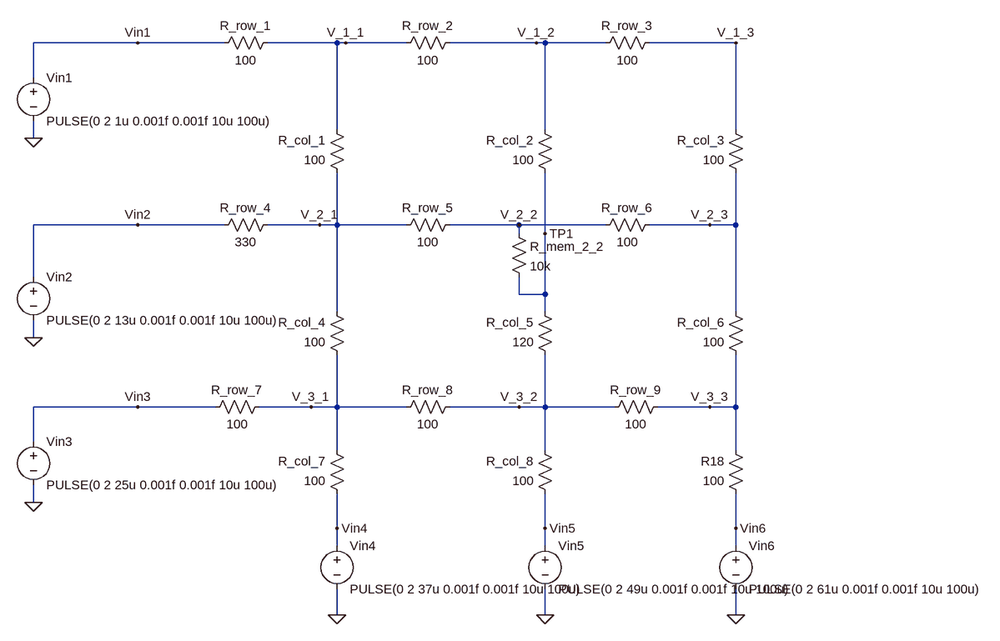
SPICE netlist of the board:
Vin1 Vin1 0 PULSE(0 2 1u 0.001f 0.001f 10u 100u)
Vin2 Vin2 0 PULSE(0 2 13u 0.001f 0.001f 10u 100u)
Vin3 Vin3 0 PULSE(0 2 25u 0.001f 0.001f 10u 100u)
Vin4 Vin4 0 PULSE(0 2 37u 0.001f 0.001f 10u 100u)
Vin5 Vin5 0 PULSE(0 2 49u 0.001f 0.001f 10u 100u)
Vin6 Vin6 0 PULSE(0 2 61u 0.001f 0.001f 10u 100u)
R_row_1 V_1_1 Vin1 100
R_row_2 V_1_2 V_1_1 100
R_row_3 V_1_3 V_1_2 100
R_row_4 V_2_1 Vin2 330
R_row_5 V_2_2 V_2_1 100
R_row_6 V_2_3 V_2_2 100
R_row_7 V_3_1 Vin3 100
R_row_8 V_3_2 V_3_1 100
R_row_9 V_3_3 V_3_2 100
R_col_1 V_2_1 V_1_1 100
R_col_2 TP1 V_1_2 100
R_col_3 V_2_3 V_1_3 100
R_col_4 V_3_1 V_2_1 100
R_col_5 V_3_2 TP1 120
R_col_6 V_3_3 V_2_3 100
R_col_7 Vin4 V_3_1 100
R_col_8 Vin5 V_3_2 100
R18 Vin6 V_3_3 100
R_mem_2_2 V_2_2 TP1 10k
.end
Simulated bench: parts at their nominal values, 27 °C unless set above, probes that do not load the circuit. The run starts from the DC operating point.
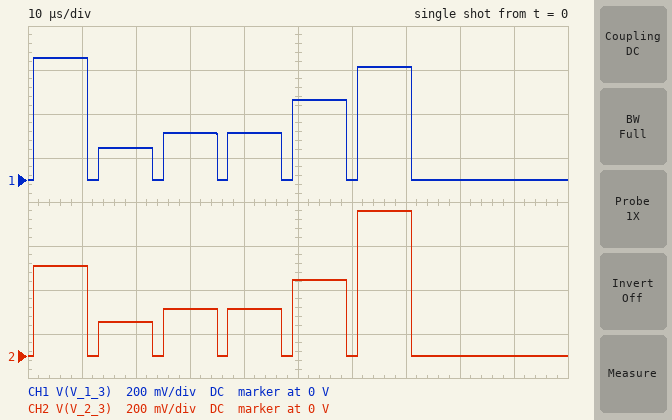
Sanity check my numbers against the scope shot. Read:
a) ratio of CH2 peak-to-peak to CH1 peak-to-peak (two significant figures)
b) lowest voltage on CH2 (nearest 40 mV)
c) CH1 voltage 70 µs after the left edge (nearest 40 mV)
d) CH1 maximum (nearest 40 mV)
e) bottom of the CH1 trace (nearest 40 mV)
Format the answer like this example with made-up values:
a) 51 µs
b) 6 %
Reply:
a) 1.2
b) 0 V
c) 520 mV
d) 560 mV
e) 0 V
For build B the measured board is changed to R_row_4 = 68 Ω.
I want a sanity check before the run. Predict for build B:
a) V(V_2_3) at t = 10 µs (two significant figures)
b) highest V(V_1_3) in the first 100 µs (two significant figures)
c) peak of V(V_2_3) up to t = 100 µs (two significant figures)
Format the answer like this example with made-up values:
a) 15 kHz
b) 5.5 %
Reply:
a) 310 mV
b) 470 mV
c) 620 mV
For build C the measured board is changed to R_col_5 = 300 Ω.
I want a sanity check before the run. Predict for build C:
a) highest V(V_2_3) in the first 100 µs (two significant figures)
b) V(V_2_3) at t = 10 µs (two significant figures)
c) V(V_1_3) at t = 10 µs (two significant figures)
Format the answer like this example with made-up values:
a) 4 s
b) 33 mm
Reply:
a) 660 mV
b) 430 mV
c) 600 mV
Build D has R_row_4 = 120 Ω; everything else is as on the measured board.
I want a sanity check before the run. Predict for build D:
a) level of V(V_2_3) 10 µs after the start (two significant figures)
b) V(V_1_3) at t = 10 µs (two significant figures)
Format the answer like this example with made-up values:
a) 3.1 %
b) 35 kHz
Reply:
a) 350 mV
b) 500 mV
